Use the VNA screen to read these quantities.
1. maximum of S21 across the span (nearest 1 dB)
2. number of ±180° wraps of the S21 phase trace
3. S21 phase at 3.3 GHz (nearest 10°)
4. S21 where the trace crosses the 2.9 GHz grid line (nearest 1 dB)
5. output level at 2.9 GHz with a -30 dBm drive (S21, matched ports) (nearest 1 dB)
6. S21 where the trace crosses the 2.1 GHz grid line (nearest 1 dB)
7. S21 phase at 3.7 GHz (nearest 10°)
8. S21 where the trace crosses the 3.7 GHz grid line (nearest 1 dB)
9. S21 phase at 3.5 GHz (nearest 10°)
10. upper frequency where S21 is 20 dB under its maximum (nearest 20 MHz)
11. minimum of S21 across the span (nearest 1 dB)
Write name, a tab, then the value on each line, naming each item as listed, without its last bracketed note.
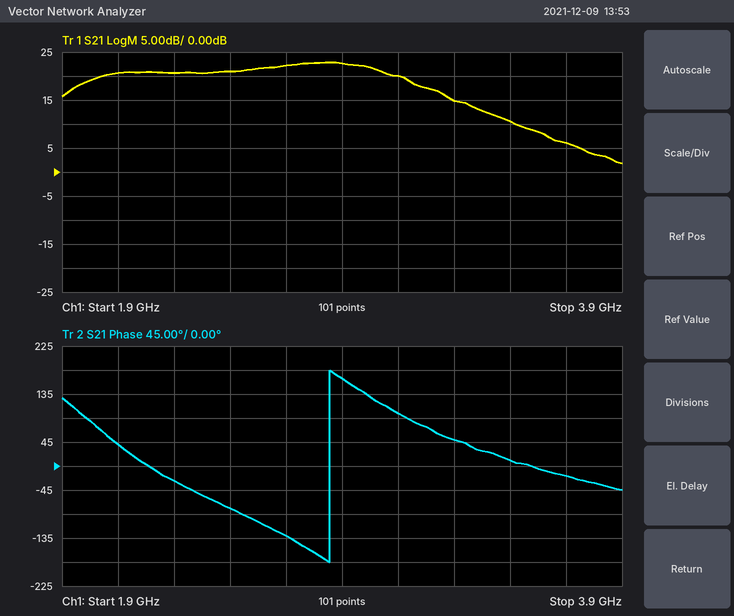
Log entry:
maximum of S21 across the span	23 dB
number of ±180° wraps of the S21 phase trace	1
S21 phase at 3.3 GHz	50°
S21 where the trace crosses the 2.9 GHz grid line	23 dB
output level at 2.9 GHz with a -30 dBm drive (S21, matched ports)	-7 dBm
S21 where the trace crosses the 2.1 GHz grid line	21 dB
S21 phase at 3.7 GHz	-20°
S21 where the trace crosses the 3.7 GHz grid line	6 dB
S21 phase at 3.5 GHz	10°
upper frequency where S21 is 20 dB under its maximum	3.86 GHz
minimum of S21 across the span	2 dB
